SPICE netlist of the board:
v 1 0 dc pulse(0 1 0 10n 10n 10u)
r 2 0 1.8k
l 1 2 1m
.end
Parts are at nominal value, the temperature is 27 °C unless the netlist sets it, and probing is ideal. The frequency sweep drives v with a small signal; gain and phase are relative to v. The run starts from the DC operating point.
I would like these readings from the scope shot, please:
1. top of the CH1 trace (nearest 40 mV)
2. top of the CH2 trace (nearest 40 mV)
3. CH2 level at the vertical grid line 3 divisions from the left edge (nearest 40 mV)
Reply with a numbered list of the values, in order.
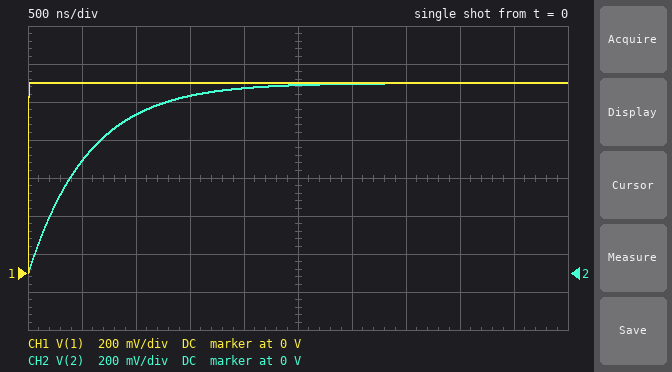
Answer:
1. 1.00 V
2. 1.00 V
3. 920 mV
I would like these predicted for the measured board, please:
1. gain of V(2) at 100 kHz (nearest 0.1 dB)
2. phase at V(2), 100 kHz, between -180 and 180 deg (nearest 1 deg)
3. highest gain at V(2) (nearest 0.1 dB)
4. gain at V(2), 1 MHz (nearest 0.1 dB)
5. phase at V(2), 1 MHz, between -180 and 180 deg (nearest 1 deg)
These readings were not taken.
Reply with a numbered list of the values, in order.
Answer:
1. -0.5 dB
2. -19 deg
3. 0 dB
4. -11.2 dB
5. -74 deg
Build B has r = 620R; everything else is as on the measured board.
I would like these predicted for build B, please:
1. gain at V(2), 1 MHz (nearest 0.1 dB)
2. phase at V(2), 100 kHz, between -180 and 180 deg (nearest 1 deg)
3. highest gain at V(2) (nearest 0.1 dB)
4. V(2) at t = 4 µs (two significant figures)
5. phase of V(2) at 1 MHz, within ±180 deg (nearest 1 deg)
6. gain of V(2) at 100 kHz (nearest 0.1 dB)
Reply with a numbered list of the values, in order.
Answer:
1. -20.2 dB
2. -45 deg
3. 0 dB
4. 920 mV
5. -84 deg
6. -3.1 dB
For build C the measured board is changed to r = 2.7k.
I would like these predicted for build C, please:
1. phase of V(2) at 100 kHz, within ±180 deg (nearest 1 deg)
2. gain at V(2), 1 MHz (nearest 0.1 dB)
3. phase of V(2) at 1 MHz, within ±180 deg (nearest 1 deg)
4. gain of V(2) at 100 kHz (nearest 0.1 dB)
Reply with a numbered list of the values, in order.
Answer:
1. -13 deg
2. -8.1 dB
3. -67 deg
4. -0.2 dB
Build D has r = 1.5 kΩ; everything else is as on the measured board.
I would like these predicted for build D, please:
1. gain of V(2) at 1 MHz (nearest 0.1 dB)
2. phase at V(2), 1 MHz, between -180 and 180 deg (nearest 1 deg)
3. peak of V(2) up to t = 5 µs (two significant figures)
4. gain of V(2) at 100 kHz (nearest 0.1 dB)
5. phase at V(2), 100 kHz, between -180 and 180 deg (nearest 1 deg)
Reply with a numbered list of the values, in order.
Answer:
1. -12.7 dB
2. -77 deg
3. 1.0 V
4. -0.7 dB
5. -23 deg
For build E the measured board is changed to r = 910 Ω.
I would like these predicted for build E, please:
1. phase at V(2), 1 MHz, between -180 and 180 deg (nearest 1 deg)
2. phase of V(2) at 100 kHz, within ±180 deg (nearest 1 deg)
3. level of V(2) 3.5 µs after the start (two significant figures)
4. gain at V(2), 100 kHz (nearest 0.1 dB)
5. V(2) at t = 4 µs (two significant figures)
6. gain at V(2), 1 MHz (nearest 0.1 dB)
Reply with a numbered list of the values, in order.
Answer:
1. -82 deg
2. -35 deg
3. 960 mV
4. -1.7 dB
5. 970 mV
6. -16.9 dB
